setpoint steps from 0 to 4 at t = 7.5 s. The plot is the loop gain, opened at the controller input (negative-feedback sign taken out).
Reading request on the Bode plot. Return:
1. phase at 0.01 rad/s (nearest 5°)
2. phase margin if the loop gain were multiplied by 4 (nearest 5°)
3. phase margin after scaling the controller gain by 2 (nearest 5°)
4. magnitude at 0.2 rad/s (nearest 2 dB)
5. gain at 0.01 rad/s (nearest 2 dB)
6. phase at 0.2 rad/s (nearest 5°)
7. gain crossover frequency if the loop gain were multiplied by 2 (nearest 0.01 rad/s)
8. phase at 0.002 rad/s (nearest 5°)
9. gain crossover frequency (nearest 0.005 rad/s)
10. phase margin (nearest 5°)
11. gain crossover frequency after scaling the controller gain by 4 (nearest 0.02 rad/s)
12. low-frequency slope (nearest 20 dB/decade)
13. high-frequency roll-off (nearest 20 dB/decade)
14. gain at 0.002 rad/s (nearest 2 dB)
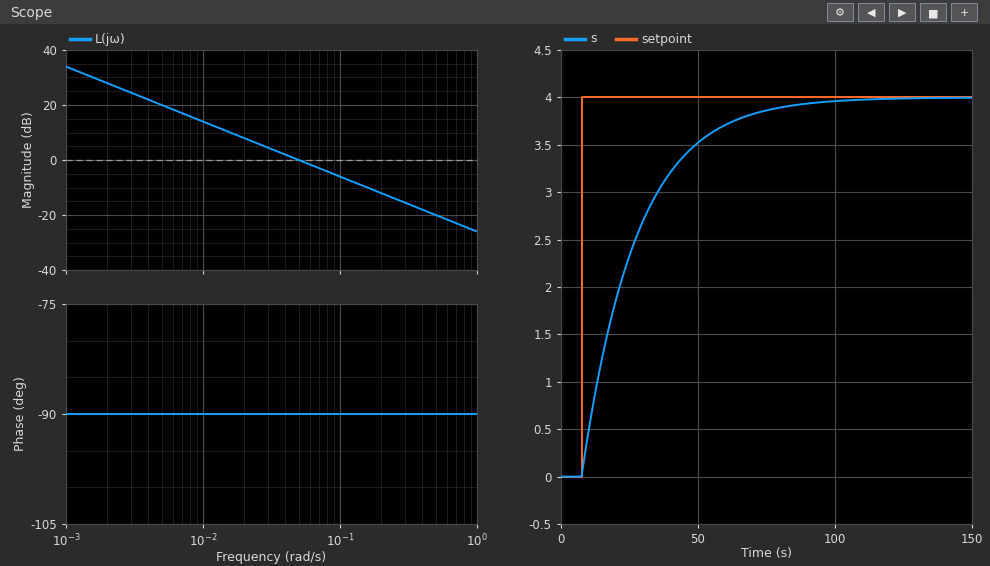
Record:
-90°
90°
90°
-12 dB
14 dB
-90°
0.10 rad/s
-90°
0.050 rad/s
90°
0.20 rad/s
-20 dB/decade
-20 dB/decade
28 dB
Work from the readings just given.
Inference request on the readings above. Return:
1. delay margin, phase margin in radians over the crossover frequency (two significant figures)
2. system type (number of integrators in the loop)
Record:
31 s
1
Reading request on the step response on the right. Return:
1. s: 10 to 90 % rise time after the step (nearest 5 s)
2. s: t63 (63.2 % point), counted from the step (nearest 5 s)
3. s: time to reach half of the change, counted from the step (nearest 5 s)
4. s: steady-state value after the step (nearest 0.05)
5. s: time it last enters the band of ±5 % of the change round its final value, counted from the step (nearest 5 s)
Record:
45 s
20 s
15 s
4.00
60 s
